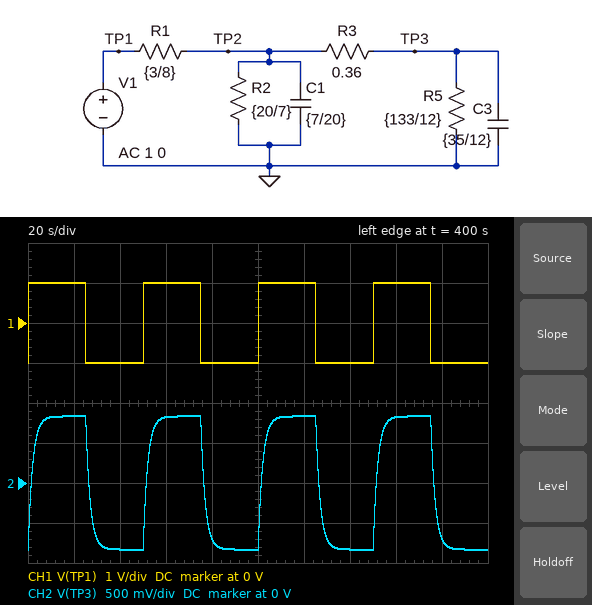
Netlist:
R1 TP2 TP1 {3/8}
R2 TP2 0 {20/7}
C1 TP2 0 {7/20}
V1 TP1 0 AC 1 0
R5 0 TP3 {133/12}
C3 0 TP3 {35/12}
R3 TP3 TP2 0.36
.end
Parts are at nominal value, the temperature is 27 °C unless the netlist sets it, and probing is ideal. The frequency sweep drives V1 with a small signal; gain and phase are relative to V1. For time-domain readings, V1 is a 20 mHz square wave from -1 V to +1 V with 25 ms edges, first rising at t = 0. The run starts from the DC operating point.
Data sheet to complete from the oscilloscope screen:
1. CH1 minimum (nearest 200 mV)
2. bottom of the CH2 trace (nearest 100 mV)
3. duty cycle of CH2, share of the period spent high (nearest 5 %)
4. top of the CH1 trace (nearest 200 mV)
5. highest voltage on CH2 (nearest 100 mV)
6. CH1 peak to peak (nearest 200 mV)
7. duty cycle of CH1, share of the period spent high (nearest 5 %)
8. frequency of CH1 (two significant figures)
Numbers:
-1.0 V
-800 mV
50 %
1.0 V
800 mV
2.0 V
50 %
20 mHz
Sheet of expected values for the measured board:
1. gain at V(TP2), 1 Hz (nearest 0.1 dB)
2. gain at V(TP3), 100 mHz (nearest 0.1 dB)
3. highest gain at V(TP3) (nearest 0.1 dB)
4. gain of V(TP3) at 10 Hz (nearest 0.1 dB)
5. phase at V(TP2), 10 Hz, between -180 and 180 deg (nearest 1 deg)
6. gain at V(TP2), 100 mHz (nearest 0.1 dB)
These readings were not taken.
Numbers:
-7.5 dB
-5.6 dB
-1.6 dB
-55.0 dB
-75 deg
-3.8 dB
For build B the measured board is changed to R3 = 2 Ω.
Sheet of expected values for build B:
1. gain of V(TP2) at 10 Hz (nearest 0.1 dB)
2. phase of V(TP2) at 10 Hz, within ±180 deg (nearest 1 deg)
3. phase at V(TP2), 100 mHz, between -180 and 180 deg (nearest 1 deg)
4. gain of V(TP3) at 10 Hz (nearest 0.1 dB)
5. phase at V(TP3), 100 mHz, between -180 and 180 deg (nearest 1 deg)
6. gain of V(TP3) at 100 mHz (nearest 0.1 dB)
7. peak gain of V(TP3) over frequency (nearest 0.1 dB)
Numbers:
-18.4 dB
-81 deg
-6 deg
-69.7 dB
-78 deg
-14.1 dB
-2.7 dB
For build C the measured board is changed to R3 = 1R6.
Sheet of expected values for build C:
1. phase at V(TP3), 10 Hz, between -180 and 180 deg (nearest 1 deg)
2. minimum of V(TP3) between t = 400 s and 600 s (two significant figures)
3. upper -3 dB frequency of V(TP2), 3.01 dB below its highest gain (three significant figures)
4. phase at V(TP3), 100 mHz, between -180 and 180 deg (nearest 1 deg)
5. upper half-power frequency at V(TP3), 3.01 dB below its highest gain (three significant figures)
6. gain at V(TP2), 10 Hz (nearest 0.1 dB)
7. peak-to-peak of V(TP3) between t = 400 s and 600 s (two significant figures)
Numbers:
-170 deg
-740 mV
1.10 Hz
-75 deg
33.0 mHz
-18.4 dB
1.5 V
